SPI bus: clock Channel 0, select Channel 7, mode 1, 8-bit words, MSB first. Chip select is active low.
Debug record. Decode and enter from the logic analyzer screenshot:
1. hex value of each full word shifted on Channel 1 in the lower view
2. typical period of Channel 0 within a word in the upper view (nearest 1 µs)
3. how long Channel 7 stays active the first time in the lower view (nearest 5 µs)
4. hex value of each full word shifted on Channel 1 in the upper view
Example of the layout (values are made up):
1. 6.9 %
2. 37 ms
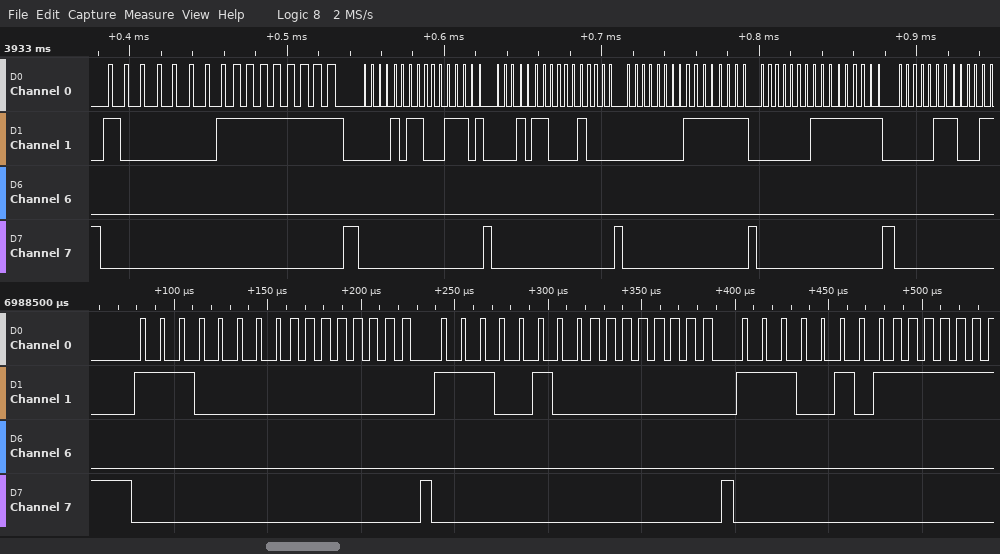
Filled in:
1. E0, 00, E4, 00, E5
2. 5 µs
3. 155 µs
4. 81, FF, 0B, 1D, 16, 10, 00, FF, 01, FF, 07
